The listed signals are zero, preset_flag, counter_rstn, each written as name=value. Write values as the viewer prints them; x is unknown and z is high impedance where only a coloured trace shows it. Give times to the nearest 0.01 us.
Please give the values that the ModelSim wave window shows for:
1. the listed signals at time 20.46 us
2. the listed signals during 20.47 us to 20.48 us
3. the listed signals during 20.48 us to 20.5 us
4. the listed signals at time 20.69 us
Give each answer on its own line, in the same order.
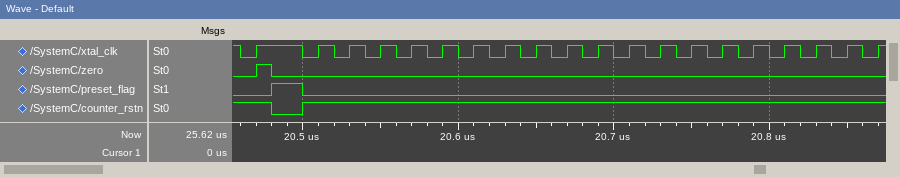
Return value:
zero=0, preset_flag=0, counter_rstn=1
zero=1, preset_flag=0, counter_rstn=1
zero=0, preset_flag=1, counter_rstn=0
zero=0, preset_flag=0, counter_rstn=1
